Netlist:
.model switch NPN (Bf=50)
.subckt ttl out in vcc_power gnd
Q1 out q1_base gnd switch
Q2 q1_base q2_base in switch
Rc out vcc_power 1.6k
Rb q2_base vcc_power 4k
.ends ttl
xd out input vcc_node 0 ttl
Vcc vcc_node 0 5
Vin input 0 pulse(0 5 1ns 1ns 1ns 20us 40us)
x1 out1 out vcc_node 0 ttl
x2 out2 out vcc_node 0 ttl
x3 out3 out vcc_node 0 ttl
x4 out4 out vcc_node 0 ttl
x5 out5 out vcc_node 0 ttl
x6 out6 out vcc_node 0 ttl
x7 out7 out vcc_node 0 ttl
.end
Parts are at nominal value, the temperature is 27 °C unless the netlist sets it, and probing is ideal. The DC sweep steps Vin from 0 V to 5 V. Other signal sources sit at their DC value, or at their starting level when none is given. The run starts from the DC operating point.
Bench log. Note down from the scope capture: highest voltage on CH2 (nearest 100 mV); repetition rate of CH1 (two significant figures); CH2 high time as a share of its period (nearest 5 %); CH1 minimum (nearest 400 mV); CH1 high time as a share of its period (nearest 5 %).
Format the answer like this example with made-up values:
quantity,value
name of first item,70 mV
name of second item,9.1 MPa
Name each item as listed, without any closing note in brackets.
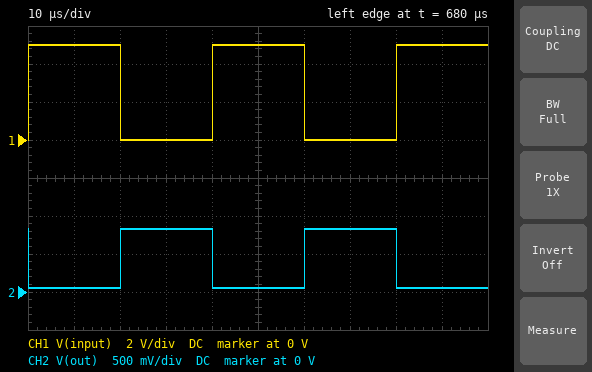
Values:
quantity,value
highest voltage on CH2,800 mV
repetition rate of CH1,25 kHz
CH2 high time as a share of its period,50 %
CH1 minimum,0 V
CH1 high time as a share of its period,50 %
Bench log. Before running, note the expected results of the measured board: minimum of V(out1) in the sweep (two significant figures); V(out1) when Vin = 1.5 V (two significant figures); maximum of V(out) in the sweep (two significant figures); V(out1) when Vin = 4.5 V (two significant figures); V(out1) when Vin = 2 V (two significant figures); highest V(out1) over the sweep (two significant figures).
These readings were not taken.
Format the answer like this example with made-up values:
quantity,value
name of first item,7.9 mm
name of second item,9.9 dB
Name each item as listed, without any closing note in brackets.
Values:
quantity,value
minimum of V(out1) in the sweep,40 mV
V(out1) when Vin = 1.5 V,5.0 V
maximum of V(out) in the sweep,830 mV
V(out1) when Vin = 4.5 V,5.0 V
V(out1) when Vin = 2 V,5.0 V
highest V(out1) over the sweep,5.0 V
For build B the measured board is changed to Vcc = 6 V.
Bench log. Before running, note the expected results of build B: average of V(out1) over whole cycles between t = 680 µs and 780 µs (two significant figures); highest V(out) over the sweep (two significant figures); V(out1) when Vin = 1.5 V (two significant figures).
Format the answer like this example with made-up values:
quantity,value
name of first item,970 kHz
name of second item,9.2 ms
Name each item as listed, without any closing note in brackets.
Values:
quantity,value
average of V(out1) over whole cycles between t = 680 µs and 780 µs,3.0 V
highest V(out) over the sweep,840 mV
V(out1) when Vin = 1.5 V,6.0 V
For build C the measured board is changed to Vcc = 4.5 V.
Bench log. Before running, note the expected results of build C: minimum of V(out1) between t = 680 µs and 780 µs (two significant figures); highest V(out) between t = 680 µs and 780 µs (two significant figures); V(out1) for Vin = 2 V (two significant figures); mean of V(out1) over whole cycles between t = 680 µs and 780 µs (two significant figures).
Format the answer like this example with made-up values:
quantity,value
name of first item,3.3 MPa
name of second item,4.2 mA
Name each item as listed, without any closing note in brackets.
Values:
quantity,value
minimum of V(out1) between t = 680 µs and 780 µs,41 mV
highest V(out) between t = 680 µs and 780 µs,830 mV
V(out1) for Vin = 2 V,4.5 V
mean of V(out1) over whole cycles between t = 680 µs and 780 µs,2.3 V
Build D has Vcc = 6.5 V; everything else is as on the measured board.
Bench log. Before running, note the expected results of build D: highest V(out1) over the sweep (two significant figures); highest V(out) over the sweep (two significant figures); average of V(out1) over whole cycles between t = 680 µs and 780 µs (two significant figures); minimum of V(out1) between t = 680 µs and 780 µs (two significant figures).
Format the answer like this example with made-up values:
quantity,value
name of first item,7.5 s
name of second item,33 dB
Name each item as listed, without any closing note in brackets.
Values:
quantity,value
highest V(out1) over the sweep,6.5 V
highest V(out) over the sweep,840 mV
average of V(out1) over whole cycles between t = 680 µs and 780 µs,3.3 V
minimum of V(out1) between t = 680 µs and 780 µs,39 mV
